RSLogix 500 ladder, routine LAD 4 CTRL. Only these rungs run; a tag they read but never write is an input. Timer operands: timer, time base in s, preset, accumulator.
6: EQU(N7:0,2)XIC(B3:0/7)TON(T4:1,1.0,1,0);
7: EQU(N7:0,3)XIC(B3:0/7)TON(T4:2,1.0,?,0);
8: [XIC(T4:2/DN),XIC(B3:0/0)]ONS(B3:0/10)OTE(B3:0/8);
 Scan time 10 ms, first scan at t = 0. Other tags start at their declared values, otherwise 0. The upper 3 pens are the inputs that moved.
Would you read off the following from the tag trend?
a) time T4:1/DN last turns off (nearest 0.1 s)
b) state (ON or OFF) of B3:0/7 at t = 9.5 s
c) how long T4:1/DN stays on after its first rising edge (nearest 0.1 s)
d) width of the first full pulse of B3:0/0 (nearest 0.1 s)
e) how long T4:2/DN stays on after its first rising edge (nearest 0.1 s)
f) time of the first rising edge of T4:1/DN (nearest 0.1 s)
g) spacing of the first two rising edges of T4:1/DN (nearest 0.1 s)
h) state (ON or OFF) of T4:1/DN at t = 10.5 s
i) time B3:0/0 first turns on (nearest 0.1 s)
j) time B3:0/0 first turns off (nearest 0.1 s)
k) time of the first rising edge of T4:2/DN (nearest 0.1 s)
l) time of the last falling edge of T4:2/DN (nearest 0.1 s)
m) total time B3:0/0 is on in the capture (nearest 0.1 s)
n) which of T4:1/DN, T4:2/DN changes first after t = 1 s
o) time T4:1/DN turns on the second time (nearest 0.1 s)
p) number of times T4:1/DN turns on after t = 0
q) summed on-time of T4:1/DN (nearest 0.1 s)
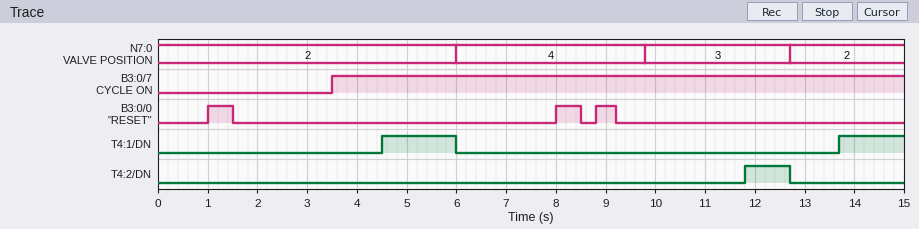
6.0 s
ON
1.5 s
0.5 s
0.9 s
4.5 s
9.2 s
OFF
1.0 s
1.5 s
11.8 s
12.7 s
1.4 s
T4:1/DN
13.7 s
2
2.8 s
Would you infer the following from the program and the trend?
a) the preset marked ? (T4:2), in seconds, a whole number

2 s
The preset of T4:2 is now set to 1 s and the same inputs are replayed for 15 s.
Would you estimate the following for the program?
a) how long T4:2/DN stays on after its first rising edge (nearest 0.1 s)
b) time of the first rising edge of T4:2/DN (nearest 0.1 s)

1.9 s
10.8 s
